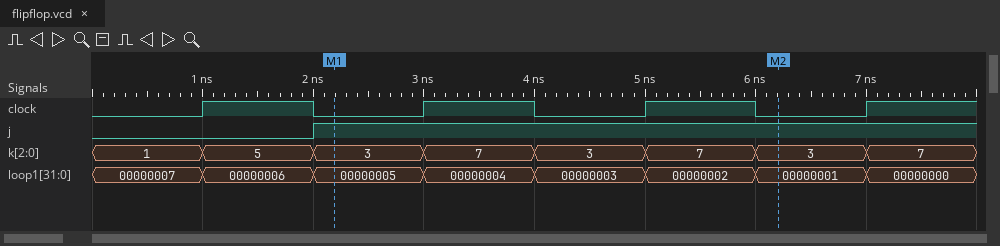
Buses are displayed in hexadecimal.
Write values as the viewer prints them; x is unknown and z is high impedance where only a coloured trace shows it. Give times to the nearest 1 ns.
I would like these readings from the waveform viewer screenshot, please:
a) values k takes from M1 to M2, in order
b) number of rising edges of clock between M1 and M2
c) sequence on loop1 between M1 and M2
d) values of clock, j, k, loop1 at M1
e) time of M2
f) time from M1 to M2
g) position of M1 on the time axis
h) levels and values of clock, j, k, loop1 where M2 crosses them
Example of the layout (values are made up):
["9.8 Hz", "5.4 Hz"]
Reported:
["3, 7, 3, 7, 3", "2", "00000005, 00000004, 00000003, 00000002, 00000001", "clock=0, j=1, k=3, loop1=00000005", "6 ns", "4 ns", "2 ns", "clock=0, j=1, k=3, loop1=00000001"]
